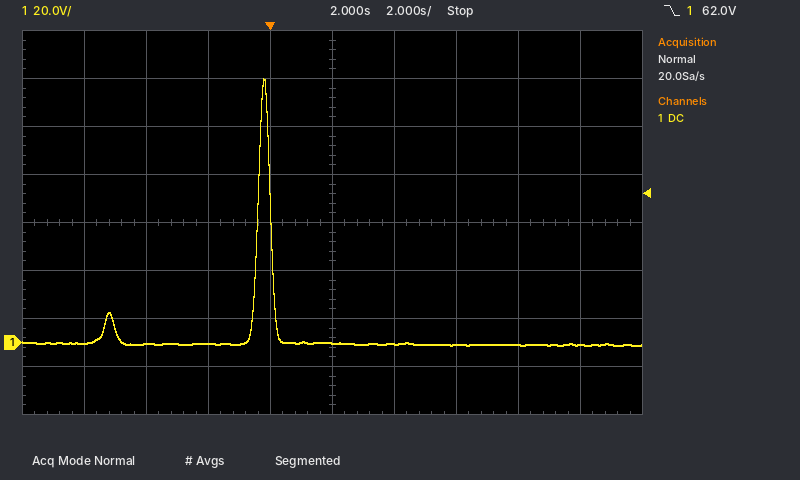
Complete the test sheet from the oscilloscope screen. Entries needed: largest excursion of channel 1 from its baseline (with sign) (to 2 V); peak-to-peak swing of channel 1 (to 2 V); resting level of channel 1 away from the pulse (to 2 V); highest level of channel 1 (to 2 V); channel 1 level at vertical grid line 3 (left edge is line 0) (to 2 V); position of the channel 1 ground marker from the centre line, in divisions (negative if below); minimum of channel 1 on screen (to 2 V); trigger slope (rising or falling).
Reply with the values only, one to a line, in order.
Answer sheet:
+110 V
112 V
0 V
110 V
0 V
-2.5 div
-2 V
falling
